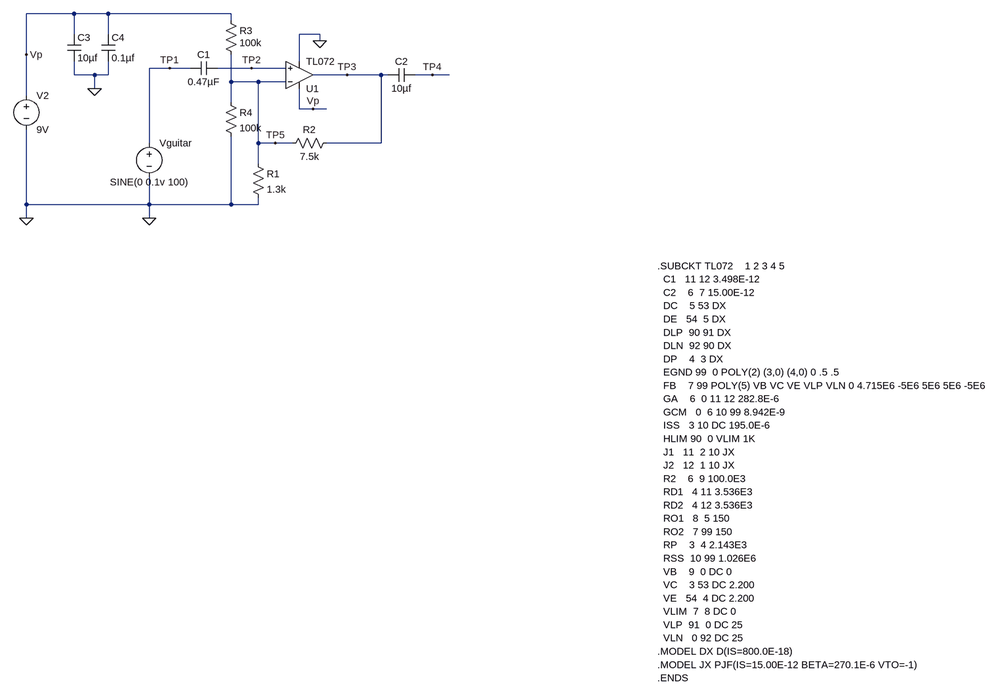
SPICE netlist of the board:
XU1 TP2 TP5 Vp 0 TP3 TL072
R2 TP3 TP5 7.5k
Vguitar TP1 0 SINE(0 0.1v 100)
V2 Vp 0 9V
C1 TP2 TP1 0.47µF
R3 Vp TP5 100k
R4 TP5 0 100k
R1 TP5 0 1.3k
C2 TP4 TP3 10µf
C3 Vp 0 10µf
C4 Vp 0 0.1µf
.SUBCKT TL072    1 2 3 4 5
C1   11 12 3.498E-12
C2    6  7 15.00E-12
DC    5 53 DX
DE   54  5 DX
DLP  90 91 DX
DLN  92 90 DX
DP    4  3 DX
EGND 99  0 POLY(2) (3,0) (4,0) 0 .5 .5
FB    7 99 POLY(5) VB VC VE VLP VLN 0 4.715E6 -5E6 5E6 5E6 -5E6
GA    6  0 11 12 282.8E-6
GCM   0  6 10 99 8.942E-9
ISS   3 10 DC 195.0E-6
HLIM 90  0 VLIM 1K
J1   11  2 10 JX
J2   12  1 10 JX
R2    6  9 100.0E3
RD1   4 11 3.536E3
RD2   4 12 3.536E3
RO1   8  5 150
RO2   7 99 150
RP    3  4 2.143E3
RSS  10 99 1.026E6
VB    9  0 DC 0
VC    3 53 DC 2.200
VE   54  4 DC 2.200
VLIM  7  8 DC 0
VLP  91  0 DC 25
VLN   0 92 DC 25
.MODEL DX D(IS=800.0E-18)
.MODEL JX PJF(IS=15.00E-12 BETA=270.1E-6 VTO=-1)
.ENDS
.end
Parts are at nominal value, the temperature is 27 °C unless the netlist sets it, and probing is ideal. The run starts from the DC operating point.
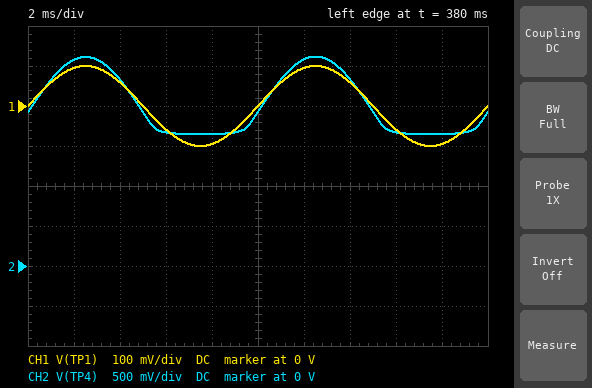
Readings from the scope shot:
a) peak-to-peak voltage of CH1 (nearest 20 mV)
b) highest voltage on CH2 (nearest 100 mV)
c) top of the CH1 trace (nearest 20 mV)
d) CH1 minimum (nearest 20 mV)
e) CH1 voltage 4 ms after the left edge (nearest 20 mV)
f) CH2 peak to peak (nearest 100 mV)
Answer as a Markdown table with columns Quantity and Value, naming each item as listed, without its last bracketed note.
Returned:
| Quantity | Value |
|---|---|
| peak-to-peak voltage of CH1 | 200 mV |
| highest voltage on CH2 | 2.6 V |
| top of the CH1 trace | 100 mV |
| CH1 minimum | -100 mV |
| CH1 voltage 4 ms after the left edge | 60 mV |
| CH2 peak to peak | 1.0 V |
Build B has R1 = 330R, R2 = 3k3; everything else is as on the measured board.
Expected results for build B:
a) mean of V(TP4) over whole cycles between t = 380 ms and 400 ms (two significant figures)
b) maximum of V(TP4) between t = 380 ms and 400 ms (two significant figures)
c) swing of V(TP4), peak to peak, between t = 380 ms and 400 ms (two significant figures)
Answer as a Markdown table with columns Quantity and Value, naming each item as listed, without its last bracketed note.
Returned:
| Quantity | Value |
|---|---|
| mean of V(TP4) over whole cycles between t = 380 ms and 400 ms | 3.8 V |
| maximum of V(TP4) between t = 380 ms and 400 ms | 4.9 V |
| swing of V(TP4), peak to peak, between t = 380 ms and 400 ms | 2.2 V |
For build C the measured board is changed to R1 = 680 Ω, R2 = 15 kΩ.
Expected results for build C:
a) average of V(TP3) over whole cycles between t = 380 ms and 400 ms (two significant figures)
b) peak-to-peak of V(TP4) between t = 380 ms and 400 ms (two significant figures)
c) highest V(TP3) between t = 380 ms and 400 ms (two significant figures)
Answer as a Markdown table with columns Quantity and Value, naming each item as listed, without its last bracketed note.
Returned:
| Quantity | Value |
|---|---|
| average of V(TP3) over whole cycles between t = 380 ms and 400 ms | 6.6 V |
| peak-to-peak of V(TP4) between t = 380 ms and 400 ms | 2.4 V |
| highest V(TP3) between t = 380 ms and 400 ms | 7.4 V |
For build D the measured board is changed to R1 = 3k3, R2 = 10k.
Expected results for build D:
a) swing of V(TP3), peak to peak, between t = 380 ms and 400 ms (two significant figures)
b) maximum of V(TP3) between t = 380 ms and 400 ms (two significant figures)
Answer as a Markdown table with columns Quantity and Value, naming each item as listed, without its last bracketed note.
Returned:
| Quantity | Value |
|---|---|
| swing of V(TP3), peak to peak, between t = 380 ms and 400 ms | 24 mV |
| maximum of V(TP3) between t = 380 ms and 400 ms | 1.6 V |
